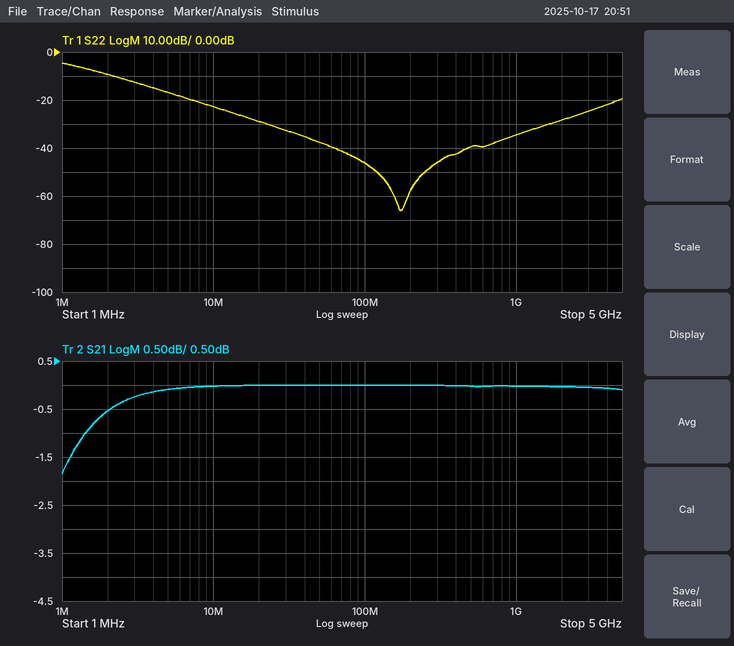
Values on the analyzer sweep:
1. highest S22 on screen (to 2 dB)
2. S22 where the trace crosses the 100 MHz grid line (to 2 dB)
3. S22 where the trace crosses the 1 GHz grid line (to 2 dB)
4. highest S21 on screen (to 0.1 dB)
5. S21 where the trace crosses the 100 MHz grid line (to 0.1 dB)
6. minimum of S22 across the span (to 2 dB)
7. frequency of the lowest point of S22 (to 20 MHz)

-4 dB
-46 dB
-34 dB
0.0 dB
0.0 dB
-66 dB
180 MHz
